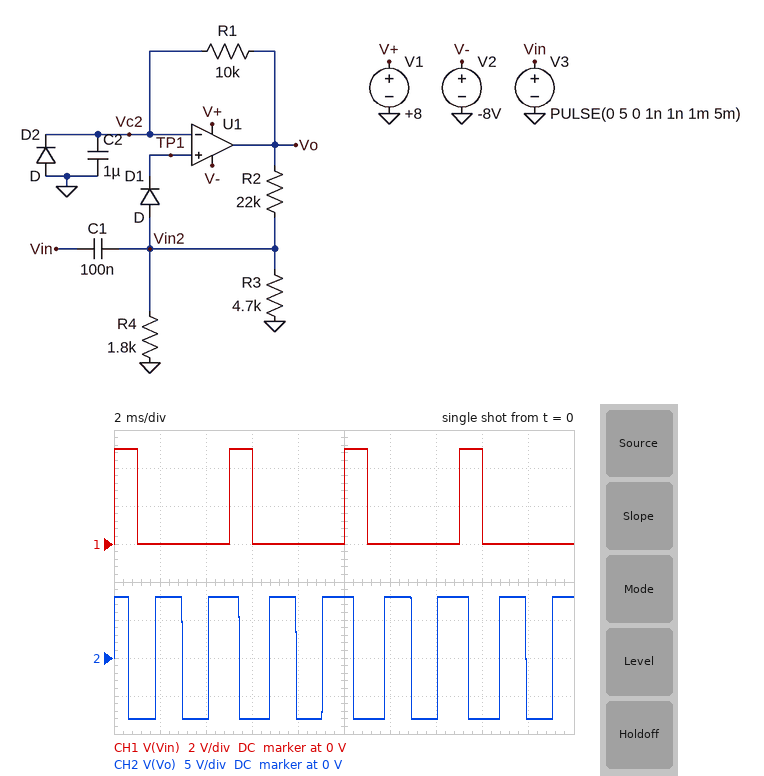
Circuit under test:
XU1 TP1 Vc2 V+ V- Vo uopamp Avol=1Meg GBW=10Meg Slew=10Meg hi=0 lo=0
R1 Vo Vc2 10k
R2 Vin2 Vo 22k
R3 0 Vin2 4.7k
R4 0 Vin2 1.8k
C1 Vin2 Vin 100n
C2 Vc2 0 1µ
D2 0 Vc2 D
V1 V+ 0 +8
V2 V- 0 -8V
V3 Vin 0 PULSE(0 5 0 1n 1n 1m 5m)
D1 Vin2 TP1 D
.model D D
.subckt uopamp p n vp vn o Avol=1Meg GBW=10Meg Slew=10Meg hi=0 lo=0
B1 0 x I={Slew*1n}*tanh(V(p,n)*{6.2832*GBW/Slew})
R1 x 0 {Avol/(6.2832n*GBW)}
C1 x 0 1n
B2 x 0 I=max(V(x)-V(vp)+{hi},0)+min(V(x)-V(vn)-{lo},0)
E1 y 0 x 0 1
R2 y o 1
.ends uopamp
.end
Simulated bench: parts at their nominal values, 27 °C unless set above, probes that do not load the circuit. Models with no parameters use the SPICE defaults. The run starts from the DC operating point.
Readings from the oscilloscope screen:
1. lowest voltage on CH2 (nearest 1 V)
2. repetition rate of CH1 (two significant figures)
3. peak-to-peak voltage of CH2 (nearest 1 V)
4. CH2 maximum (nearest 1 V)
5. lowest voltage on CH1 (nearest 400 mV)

-8 V
200 Hz
16 V
8 V
0 V
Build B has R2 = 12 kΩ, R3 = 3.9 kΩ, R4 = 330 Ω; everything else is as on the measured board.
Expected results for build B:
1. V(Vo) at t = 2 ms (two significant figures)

-8.0 V
